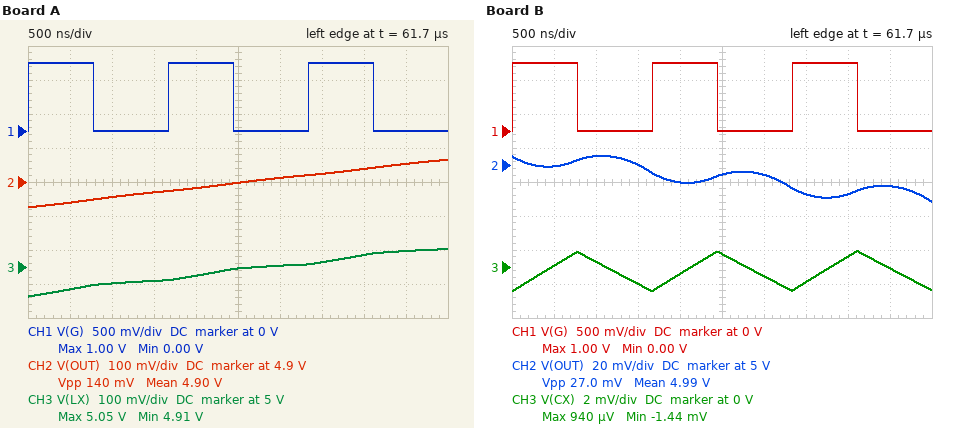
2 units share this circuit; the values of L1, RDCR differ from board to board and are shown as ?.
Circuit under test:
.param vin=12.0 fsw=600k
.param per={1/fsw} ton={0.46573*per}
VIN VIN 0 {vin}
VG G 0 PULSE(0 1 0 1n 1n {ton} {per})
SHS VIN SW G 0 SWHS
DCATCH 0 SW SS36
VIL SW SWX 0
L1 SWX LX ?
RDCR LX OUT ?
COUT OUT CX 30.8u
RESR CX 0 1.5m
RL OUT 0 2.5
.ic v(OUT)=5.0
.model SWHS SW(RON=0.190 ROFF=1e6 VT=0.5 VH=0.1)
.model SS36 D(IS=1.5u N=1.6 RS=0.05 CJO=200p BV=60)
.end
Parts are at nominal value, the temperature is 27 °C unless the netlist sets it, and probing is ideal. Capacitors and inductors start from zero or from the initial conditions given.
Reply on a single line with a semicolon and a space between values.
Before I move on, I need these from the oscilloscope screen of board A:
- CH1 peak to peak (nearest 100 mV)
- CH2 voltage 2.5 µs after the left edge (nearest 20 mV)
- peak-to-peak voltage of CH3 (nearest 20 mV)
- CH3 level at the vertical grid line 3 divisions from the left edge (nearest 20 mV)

1.0 V; 4.90 V; 140 mV; 4.96 V
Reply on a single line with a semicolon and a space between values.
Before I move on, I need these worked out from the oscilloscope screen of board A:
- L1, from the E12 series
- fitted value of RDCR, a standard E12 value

15 µH; 0.033 Ω
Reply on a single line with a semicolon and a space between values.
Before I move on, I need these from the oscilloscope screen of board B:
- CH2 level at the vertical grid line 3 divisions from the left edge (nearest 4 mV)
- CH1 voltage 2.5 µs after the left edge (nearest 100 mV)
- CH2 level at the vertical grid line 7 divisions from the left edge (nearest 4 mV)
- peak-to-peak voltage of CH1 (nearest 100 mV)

5.000 V; 0 V; 4.984 V; 1.0 V
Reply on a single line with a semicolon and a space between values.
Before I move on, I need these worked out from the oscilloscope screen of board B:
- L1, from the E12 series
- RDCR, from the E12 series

3.3 µH; 0.033 Ω
